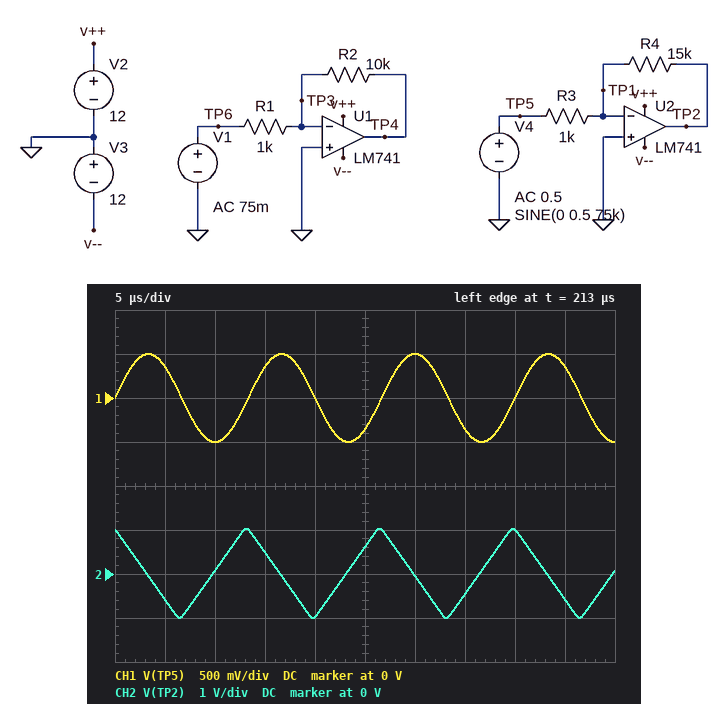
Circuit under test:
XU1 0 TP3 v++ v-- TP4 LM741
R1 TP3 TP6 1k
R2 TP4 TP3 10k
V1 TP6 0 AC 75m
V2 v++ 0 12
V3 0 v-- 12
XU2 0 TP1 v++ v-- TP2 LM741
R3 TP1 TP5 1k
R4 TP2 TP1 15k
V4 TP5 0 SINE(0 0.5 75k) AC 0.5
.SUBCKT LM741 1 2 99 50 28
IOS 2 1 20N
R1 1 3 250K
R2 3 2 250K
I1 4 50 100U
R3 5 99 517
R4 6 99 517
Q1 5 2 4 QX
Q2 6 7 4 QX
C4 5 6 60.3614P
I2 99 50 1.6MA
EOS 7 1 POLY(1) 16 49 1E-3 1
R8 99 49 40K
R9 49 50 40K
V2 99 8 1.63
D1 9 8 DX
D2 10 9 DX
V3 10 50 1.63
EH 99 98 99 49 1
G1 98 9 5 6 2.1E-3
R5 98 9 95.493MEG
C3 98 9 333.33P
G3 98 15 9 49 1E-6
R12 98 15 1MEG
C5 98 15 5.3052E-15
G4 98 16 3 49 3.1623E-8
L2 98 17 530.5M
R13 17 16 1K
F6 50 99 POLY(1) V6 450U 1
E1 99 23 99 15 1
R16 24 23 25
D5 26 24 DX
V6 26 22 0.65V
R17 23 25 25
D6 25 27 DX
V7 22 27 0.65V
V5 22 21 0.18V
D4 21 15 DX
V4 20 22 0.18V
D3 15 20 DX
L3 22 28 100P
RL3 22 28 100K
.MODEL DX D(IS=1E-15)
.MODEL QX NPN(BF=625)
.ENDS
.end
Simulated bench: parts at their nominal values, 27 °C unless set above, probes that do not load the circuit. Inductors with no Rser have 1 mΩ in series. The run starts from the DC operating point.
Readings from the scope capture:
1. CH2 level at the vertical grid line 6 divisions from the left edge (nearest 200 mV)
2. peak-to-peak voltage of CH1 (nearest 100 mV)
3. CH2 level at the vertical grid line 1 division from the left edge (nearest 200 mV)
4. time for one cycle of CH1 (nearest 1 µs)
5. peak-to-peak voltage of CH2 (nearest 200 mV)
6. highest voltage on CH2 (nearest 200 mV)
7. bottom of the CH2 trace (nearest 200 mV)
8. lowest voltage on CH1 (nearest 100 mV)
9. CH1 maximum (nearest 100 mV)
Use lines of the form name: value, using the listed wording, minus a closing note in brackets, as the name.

CH2 level at the vertical grid line 6 divisions from the left edge: 0 V
peak-to-peak voltage of CH1: 1.0 V
CH2 level at the vertical grid line 1 division from the left edge: -600 mV
time for one cycle of CH1: 13 µs
peak-to-peak voltage of CH2: 2.0 V
highest voltage on CH2: 1.0 V
bottom of the CH2 trace: -1.0 V
lowest voltage on CH1: -500 mV
CH1 maximum: 500 mV
